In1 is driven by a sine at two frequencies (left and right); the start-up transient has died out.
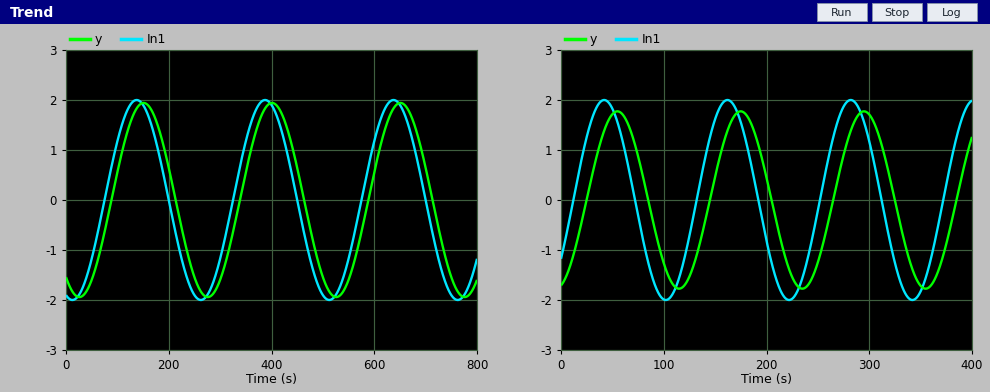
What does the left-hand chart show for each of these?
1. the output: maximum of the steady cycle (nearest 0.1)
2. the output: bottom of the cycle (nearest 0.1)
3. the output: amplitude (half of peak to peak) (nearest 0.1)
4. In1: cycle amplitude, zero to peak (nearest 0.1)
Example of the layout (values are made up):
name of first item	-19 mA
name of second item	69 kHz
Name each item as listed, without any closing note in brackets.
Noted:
the output: maximum of the steady cycle	1.9
the output: bottom of the cycle	-1.9
the output: amplitude (half of peak to peak)	1.9
In1: cycle amplitude, zero to peak	2.0
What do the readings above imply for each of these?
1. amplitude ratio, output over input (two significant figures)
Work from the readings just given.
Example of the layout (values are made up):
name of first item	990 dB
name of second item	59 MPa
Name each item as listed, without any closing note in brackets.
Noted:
amplitude ratio, output over input	0.95
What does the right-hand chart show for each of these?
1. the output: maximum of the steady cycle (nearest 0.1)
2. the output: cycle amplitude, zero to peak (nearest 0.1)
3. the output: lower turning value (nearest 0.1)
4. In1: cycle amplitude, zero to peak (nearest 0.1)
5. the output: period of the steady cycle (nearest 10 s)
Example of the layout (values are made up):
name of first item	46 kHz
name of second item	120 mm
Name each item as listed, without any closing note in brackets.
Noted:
the output: maximum of the steady cycle	1.8
the output: cycle amplitude, zero to peak	1.8
the output: lower turning value	-1.8
In1: cycle amplitude, zero to peak	2.0
the output: period of the steady cycle	120 s
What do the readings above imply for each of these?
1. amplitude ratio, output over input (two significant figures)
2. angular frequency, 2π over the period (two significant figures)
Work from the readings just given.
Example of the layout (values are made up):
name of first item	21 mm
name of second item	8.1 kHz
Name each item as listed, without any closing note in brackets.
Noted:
amplitude ratio, output over input	0.90
angular frequency, 2π over the period	0.052 rad/s
